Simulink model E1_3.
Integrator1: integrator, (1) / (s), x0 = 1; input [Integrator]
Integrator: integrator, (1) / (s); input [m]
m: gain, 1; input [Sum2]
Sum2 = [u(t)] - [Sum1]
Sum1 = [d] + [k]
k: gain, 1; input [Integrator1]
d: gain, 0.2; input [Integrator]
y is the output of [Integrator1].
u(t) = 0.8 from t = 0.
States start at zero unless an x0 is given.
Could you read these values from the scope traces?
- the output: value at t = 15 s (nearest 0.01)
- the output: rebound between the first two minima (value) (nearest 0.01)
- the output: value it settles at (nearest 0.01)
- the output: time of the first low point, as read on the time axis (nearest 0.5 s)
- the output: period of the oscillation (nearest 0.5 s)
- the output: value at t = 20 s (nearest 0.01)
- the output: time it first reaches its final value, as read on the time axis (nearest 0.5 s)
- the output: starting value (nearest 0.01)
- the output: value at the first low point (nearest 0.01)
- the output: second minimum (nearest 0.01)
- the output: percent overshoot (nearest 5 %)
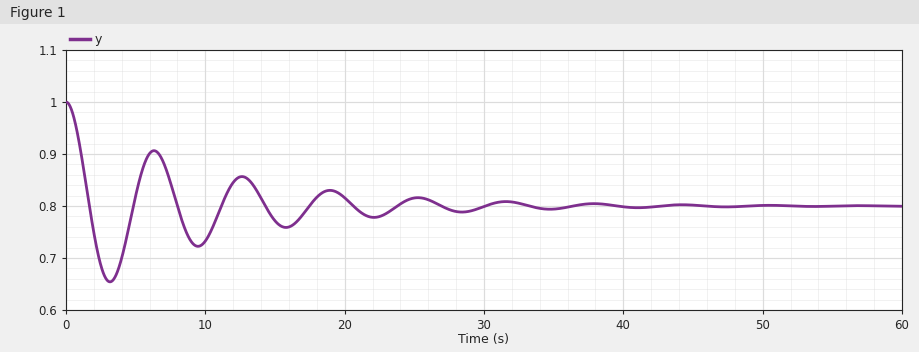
0.77
0.91
0.80
3.0 s
6.5 s
0.82
1.5 s
1.00
0.65
0.72
75 %
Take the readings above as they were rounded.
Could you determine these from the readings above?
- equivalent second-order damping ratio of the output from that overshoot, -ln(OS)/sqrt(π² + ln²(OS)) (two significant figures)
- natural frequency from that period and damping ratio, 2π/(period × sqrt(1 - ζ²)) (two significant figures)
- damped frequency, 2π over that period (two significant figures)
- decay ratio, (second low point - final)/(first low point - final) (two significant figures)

0.091
0.97 rad/s
0.97 rad/s
0.53
